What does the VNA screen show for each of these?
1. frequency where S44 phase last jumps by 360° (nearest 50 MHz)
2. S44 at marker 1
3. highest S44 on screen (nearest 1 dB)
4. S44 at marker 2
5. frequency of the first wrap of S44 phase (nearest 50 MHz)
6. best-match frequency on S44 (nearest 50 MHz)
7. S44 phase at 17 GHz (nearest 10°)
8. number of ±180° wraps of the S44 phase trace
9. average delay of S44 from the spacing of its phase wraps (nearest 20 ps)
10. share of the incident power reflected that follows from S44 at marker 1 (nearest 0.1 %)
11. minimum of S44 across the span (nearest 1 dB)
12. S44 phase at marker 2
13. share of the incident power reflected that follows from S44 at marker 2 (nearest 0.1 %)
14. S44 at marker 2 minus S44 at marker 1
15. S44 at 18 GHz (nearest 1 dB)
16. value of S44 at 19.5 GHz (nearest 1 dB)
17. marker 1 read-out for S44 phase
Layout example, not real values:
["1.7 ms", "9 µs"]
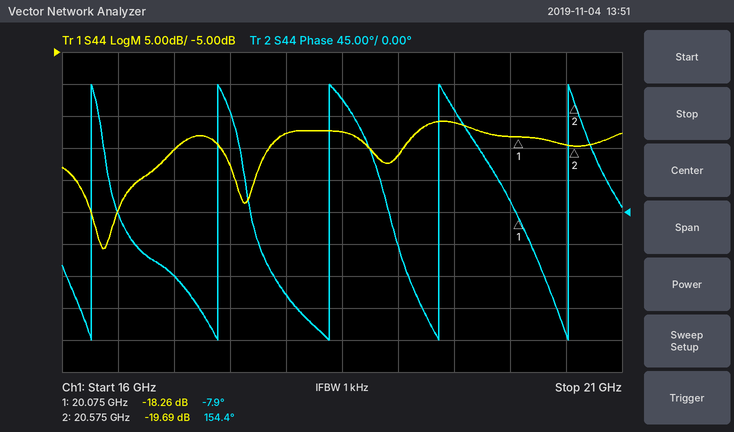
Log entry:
["20.50 GHz", "-18.26 dB", "-16 dB", "-19.69 dB", "16.25 GHz", "16.35 GHz", "-90°", "5", "940 ps", "1.5 %", "-36 dB", "154.4°", "1.1 %", "-1.43 dB", "-18 dB", "-16 dB", "-7.9°"]
